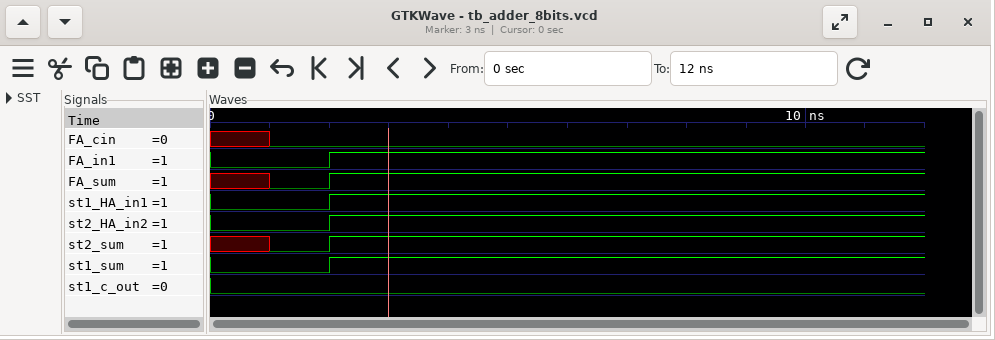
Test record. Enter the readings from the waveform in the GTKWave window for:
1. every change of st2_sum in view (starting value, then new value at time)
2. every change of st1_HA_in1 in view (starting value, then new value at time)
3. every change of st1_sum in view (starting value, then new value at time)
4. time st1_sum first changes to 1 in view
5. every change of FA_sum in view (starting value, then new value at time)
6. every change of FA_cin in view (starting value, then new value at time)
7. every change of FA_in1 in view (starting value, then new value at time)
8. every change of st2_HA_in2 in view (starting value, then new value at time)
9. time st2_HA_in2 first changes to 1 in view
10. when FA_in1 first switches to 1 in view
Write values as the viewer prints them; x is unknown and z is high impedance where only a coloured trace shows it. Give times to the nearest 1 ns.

x, 0 at 1 ns, 1 at 2 ns
0, 1 at 2 ns
0, 1 at 2 ns
2 ns
x, 0 at 1 ns, 1 at 2 ns
x, 0 at 1 ns
0, 1 at 2 ns
0, 1 at 2 ns
2 ns
2 ns
